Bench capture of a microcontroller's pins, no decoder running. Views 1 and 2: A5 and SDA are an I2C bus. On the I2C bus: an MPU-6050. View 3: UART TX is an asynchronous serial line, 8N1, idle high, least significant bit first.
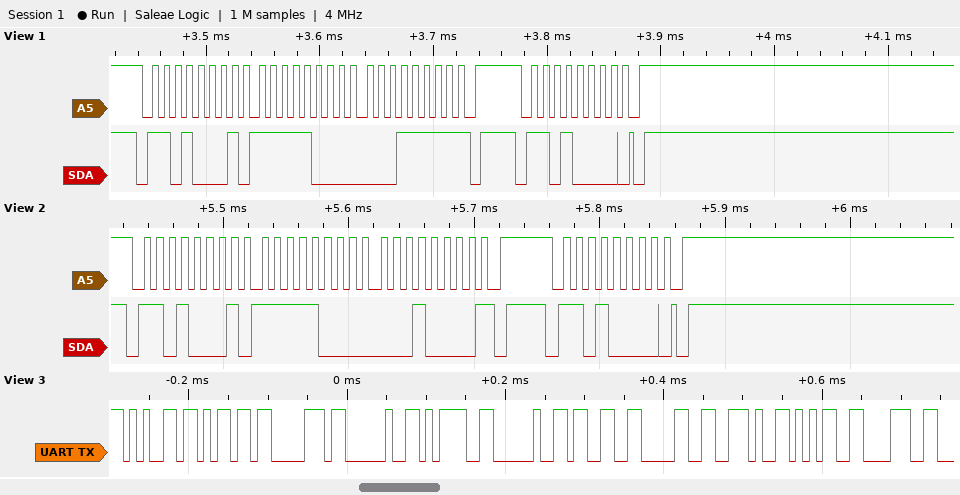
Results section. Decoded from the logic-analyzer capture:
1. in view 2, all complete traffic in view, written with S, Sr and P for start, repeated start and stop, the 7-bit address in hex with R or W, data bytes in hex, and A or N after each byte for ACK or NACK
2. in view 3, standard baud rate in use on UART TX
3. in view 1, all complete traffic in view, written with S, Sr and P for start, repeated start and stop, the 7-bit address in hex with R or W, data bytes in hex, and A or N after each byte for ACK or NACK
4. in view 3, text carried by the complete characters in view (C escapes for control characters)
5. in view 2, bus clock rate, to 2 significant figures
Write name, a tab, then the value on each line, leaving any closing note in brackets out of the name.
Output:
in view 2, all complete traffic in view, written with S, Sr and P for start, repeated start and stop, the 7-bit address in hex with R or W, data bytes in hex, and A or N after each byte for ACK or NACK	S 68R A F8 A 10 N P S 68W A P
in view 3, standard baud rate in use on UART TX	115200 baud
in view 1, all complete traffic in view, written with S, Sr and P for start, repeated start and stop, the 7-bit address in hex with R or W, data bytes in hex, and A or N after each byte for ACK or NACK	S 68R A F8 A 1F N P S 68W A P
in view 3, text carried by the complete characters in view	"emp = 30.58"
in view 2, bus clock rate, to 2 significant figures	100 kHz
